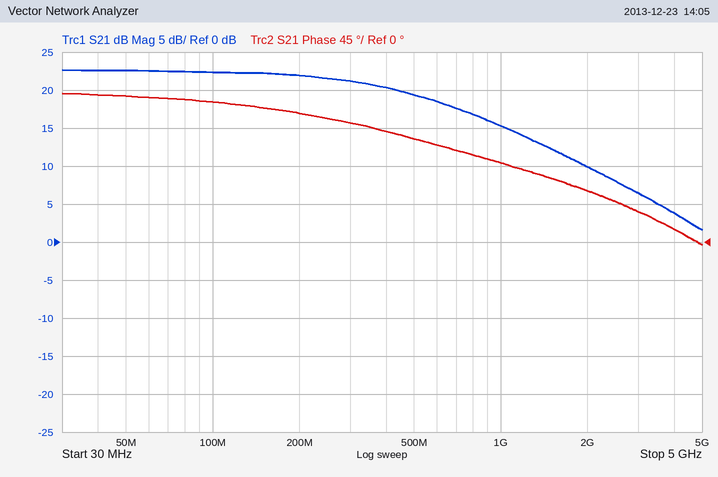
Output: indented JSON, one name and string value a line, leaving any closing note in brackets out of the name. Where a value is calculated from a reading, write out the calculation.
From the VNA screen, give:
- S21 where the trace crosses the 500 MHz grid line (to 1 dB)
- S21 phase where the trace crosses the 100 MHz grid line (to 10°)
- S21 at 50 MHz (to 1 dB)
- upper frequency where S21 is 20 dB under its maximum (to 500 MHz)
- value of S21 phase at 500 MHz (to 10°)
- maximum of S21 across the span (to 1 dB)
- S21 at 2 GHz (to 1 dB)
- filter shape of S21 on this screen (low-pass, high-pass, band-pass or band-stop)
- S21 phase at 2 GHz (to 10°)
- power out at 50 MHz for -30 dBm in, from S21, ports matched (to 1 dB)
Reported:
{
  "S21 where the trace crosses the 500 MHz grid line": "19 dB",
  "S21 phase where the trace crosses the 100 MHz grid line": "170°",
  "S21 at 50 MHz": "23 dB",
  "upper frequency where S21 is 20 dB under its maximum": "4.5 GHz",
  "value of S21 phase at 500 MHz": "120°",
  "maximum of S21 across the span": "23 dB",
  "S21 at 2 GHz": "10 dB",
  "filter shape of S21 on this screen": "low-pass",
  "S21 phase at 2 GHz": "60°",
  "power out at 50 MHz for -30 dBm in, from S21, ports matched": "-30 dBm + (23 dB) = -7 dBm"
}
